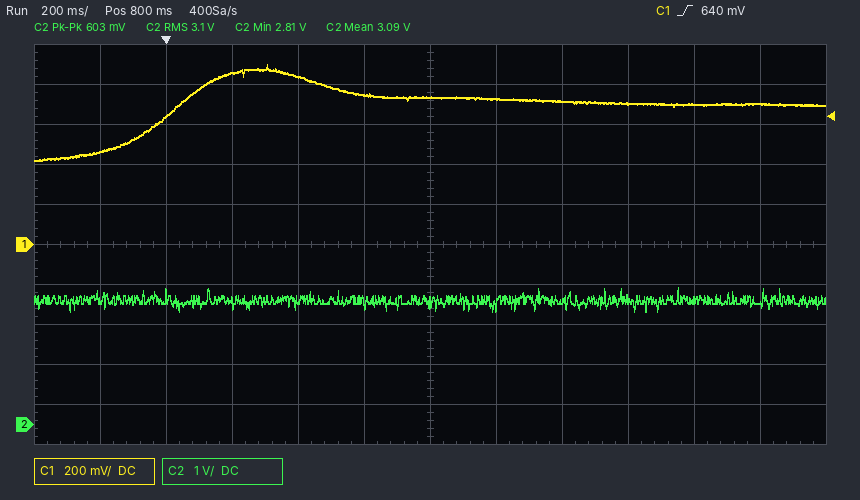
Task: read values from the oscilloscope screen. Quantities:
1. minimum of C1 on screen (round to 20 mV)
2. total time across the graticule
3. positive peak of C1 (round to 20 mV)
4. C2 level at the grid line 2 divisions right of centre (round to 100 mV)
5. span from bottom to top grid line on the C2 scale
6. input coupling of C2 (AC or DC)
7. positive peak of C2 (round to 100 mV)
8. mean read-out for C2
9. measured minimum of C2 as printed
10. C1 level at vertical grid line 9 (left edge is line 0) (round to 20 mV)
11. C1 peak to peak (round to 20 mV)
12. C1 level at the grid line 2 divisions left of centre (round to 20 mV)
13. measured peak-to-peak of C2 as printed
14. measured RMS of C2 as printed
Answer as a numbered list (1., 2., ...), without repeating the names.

1. 420 mV
2. 2.4 s
3. 900 mV
4. 3.1 V
5. 10 V
6. DC
7. 3.4 V
8. 3.09 V
9. 2.81 V
10. 700 mV
11. 480 mV
12. 840 mV
13. 603 mV
14. 3.1 V
